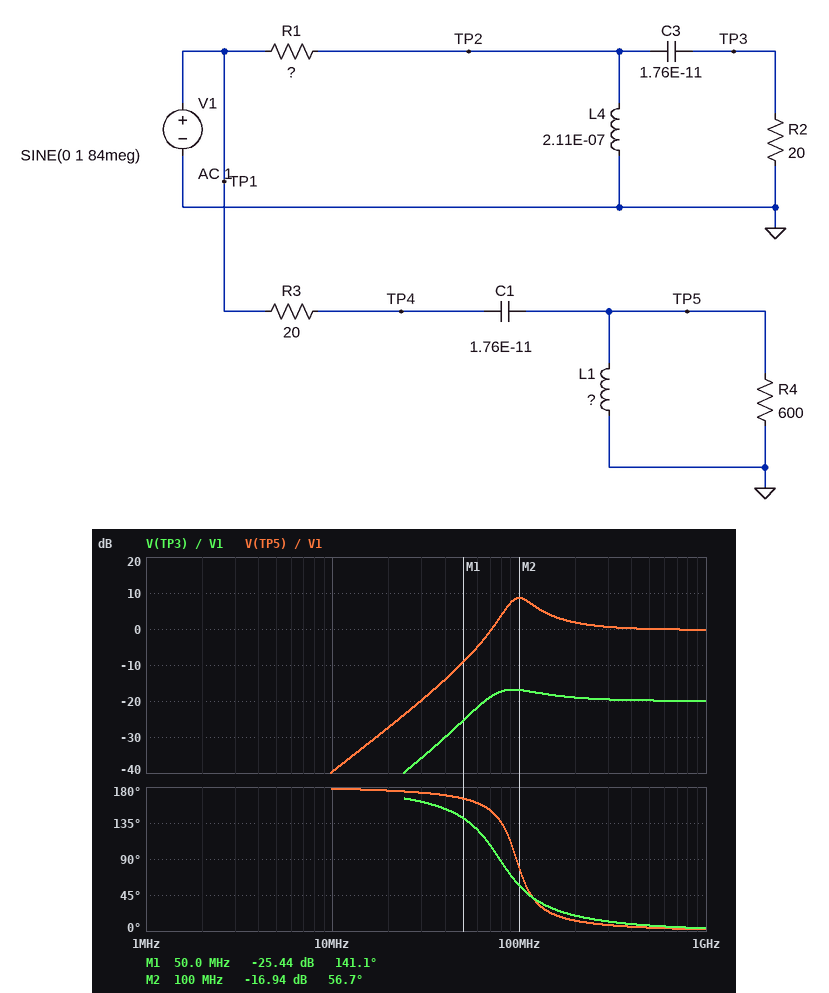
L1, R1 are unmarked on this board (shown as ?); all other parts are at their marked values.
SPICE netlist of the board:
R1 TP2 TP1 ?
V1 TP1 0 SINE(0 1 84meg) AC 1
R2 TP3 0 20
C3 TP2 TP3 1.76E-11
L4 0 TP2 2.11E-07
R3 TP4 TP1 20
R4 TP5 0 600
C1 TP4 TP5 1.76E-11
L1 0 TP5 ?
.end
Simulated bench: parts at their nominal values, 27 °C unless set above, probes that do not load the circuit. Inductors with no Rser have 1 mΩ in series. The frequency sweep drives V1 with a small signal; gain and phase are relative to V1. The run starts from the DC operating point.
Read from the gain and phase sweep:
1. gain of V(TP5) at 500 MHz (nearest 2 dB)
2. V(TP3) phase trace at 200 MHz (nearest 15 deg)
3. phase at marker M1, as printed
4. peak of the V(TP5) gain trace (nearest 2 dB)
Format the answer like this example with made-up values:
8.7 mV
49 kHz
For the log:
0 dB
15 deg
141.1 deg
8 dB
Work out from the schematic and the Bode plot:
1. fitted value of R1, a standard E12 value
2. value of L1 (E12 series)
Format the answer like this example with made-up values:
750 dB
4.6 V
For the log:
180 Ω
150 nH
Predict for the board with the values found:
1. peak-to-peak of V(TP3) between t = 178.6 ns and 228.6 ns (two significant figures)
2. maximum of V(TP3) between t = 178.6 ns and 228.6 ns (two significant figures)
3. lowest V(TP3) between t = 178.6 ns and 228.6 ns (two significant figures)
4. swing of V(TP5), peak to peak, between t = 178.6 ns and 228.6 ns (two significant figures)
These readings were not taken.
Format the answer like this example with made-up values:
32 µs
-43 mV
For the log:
280 mV
140 mV
-140 mV
3.7 V
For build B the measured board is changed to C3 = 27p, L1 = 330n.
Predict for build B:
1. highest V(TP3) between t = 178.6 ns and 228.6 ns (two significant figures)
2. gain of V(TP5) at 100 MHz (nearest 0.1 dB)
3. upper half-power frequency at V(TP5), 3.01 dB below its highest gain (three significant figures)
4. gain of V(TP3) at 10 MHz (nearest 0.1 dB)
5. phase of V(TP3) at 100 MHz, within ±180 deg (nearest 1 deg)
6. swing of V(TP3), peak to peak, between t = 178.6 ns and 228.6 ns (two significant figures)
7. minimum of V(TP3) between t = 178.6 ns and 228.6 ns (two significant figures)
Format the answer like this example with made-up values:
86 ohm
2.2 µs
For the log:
150 mV
3.8 dB
86.0 MHz
-51.9 dB
36 deg
300 mV
-150 mV
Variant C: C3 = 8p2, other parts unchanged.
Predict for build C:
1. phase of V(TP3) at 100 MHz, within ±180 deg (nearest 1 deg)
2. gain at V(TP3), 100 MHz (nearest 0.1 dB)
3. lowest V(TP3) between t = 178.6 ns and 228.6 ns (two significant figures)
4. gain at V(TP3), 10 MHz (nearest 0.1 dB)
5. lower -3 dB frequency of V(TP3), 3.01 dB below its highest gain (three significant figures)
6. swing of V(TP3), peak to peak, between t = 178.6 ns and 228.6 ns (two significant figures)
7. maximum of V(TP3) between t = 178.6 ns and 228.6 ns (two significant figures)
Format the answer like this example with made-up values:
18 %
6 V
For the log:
106 deg
-21.2 dB
-63 mV
-62.4 dB
97.7 MHz
130 mV
63 mV
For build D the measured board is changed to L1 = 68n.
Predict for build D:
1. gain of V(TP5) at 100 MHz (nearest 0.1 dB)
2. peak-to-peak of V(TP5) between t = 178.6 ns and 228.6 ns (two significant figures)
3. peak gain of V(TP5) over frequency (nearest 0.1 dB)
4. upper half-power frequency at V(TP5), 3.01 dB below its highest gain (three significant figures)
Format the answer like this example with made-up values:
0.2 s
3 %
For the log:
-1.9 dB
950 mV
7.5 dB
202 MHz
